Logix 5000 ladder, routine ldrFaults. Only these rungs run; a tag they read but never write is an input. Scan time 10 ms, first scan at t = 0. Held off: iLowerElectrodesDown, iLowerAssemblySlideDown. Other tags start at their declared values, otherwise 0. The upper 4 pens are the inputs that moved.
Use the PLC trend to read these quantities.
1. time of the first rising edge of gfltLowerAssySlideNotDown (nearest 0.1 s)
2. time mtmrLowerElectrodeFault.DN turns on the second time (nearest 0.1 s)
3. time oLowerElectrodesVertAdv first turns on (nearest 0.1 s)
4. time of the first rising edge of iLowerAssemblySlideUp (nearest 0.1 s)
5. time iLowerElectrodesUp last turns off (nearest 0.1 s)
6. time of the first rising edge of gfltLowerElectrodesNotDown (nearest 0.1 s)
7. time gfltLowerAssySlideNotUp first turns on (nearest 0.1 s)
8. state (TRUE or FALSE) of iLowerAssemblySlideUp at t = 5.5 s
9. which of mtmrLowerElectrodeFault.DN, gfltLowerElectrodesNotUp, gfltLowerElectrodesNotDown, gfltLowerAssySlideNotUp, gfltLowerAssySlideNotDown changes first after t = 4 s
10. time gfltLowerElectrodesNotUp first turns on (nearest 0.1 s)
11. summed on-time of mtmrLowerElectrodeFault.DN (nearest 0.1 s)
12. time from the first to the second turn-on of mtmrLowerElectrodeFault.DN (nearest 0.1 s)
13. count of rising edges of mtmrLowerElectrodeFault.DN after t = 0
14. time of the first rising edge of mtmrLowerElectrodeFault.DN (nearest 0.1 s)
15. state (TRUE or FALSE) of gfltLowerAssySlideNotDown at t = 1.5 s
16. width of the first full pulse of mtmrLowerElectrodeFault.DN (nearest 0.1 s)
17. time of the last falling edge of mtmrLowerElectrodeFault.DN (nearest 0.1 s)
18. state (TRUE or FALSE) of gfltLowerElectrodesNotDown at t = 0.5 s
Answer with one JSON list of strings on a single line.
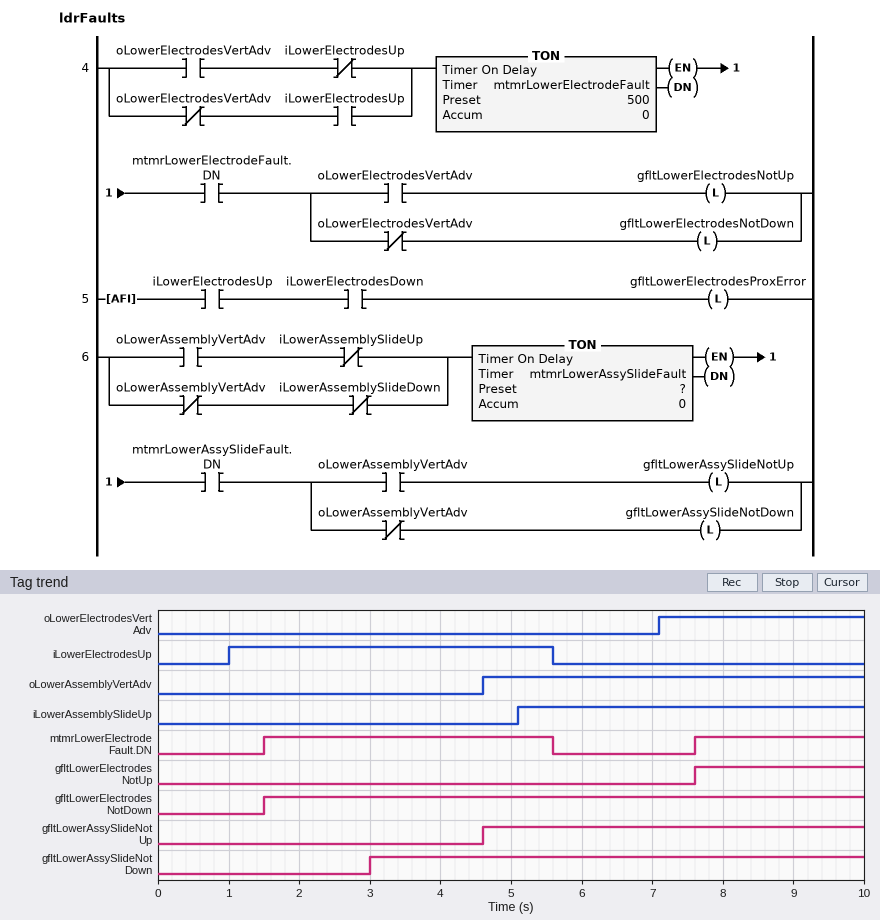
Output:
["3.0 s", "7.6 s", "7.1 s", "5.1 s", "5.6 s", "1.5 s", "4.6 s", "TRUE", "gfltLowerAssySlideNotUp", "7.6 s", "6.5 s", "6.1 s", "2", "1.5 s", "FALSE", "4.1 s", "5.6 s", "FALSE"]
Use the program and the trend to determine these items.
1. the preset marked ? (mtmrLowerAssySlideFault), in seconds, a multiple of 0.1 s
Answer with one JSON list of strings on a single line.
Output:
["3.0 s"]
